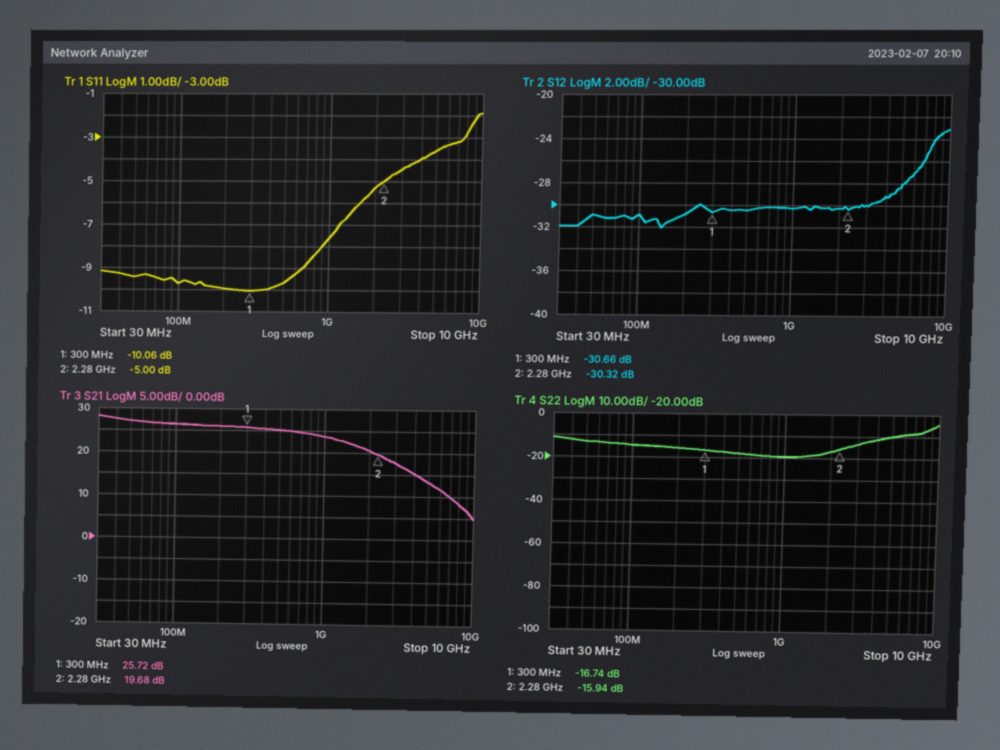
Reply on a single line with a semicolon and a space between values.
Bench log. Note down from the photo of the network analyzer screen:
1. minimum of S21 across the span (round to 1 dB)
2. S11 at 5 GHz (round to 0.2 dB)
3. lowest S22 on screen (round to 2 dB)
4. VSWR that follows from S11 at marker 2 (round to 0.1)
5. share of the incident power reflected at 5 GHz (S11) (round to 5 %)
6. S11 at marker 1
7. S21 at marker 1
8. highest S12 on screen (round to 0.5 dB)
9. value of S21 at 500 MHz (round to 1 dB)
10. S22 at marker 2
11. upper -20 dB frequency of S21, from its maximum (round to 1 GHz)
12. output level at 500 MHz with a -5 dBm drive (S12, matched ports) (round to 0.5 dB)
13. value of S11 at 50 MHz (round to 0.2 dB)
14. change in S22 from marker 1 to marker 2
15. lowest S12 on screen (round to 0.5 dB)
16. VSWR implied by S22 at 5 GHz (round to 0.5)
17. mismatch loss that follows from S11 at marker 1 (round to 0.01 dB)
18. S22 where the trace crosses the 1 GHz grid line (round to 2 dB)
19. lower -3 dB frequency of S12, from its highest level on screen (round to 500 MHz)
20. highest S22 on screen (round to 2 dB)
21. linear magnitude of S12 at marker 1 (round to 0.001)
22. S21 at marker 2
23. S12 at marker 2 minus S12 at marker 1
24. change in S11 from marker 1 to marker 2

5 dB; -3.6 dB; -20 dB; 3.6; 45 %; -10.06 dB; 25.72 dB; -23.0 dB; 25 dB; -15.94 dB; 8 GHz; -35.5 dBm; -9.4 dB; 0.80 dB; -32.0 dB; 2.0; 0.45 dB; -20 dB; 7.0 GHz; -4 dB; 0.029; 19.68 dB; 0.34 dB; 5.06 dB
